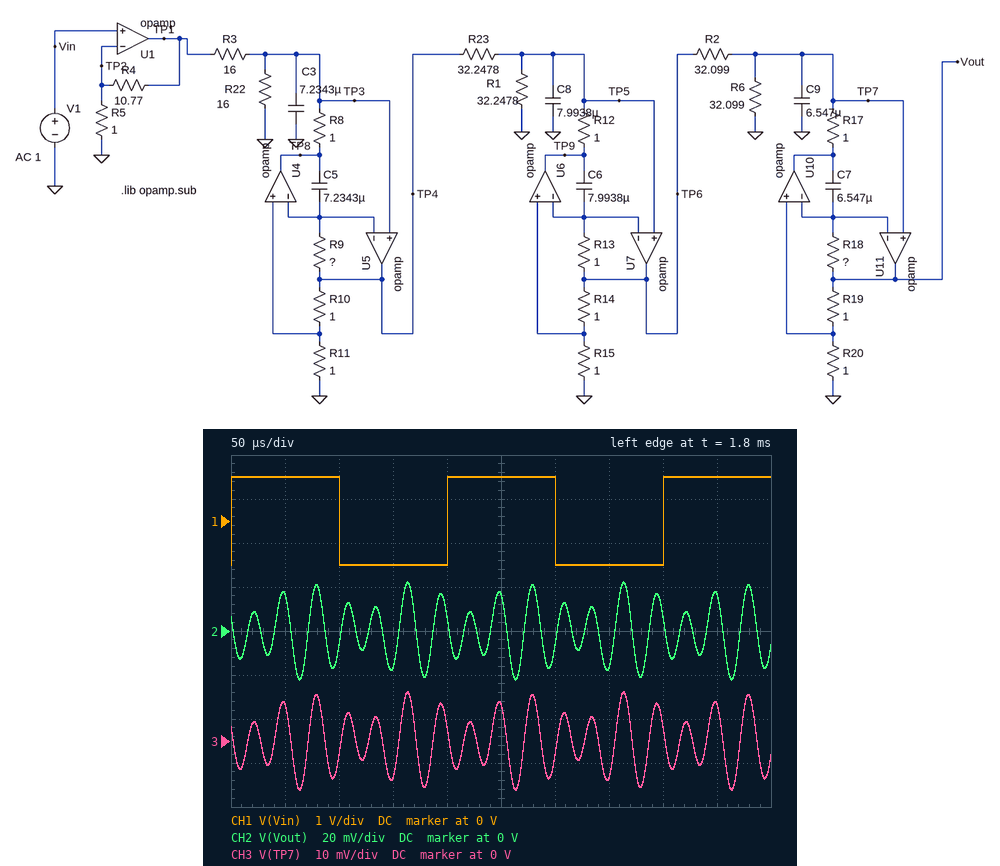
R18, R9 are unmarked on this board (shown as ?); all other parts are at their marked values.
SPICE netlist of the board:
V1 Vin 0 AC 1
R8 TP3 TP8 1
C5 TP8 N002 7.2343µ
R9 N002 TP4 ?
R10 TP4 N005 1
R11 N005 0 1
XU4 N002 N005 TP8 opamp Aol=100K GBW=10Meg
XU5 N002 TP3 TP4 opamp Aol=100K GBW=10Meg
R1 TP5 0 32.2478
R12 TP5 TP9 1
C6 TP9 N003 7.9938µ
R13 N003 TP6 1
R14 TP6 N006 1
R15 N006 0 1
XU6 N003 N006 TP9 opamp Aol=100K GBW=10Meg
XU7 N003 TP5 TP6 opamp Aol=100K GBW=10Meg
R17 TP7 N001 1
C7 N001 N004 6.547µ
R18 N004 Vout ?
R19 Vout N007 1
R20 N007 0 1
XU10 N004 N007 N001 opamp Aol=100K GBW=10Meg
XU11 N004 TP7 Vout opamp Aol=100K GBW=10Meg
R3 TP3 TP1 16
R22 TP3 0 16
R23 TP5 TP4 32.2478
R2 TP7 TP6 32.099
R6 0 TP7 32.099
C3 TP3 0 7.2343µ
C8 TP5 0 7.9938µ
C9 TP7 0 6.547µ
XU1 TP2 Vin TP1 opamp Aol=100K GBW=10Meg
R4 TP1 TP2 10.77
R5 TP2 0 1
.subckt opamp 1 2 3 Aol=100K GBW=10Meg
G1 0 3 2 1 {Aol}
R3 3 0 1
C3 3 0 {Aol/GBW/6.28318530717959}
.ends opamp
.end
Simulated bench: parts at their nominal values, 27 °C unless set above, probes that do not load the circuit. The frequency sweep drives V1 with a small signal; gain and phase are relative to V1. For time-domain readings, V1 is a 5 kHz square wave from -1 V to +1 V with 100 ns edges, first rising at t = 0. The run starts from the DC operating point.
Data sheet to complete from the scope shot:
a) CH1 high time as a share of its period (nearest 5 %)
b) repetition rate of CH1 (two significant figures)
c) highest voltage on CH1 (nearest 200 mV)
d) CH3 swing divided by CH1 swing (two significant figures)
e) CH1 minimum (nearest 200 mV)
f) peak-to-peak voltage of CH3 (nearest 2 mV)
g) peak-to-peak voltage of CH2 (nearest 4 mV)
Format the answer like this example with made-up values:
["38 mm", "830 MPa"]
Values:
["50 %", "5.0 kHz", "1.0 V", "0.011", "-1.0 V", "22 mV", "44 mV"]
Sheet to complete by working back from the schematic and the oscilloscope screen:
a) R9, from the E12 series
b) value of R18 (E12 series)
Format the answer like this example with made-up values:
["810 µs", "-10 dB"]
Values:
["0.39 Ω", "0.68 Ω"]
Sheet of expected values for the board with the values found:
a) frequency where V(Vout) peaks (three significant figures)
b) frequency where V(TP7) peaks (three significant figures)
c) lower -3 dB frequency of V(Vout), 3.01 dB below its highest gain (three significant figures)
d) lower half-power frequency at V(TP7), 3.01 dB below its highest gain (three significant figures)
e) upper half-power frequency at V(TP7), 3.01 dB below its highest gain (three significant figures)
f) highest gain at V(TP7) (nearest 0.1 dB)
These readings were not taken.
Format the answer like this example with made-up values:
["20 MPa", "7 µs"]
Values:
["29.4 kHz", "29.4 kHz", "28.6 kHz", "28.6 kHz", "30.2 kHz", "-20.2 dB"]
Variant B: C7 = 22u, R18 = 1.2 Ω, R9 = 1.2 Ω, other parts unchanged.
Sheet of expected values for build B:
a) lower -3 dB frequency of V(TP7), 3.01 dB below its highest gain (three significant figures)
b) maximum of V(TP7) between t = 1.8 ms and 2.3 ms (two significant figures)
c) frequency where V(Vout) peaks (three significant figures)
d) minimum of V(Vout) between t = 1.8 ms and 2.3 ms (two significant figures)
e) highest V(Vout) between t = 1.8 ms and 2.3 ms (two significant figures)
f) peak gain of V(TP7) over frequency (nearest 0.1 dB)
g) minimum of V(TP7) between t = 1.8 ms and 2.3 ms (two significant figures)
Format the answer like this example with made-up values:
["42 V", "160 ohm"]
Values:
["19.3 kHz", "21 mV", "19.8 kHz", "-42 mV", "42 mV", "-3.2 dB", "-21 mV"]
